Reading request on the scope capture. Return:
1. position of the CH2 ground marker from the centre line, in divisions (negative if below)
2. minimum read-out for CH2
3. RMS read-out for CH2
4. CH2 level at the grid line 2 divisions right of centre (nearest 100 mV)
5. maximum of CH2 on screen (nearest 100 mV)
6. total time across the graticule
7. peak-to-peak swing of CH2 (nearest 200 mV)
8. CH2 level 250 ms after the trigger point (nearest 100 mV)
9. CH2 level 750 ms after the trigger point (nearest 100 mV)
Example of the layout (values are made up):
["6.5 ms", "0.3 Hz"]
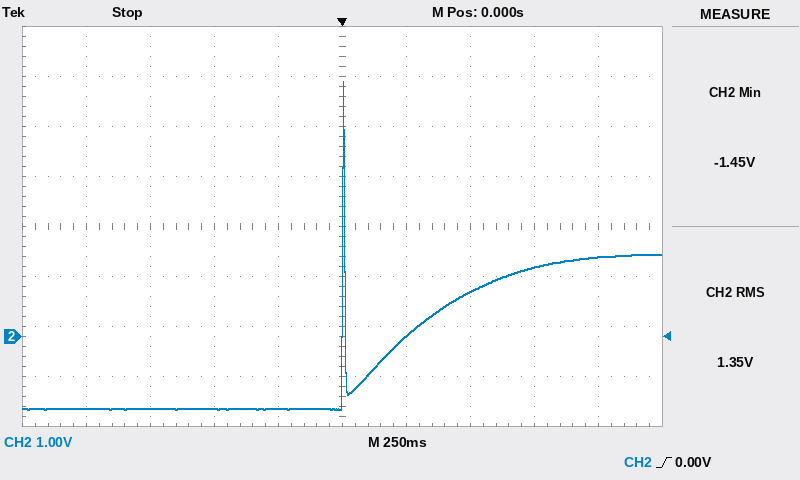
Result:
["-2.2 div", "-1.45 V", "1.35 V", "900 mV", "5.1 V", "2.5 s", "6.6 V", "0.0 V", "1.4 V"]
